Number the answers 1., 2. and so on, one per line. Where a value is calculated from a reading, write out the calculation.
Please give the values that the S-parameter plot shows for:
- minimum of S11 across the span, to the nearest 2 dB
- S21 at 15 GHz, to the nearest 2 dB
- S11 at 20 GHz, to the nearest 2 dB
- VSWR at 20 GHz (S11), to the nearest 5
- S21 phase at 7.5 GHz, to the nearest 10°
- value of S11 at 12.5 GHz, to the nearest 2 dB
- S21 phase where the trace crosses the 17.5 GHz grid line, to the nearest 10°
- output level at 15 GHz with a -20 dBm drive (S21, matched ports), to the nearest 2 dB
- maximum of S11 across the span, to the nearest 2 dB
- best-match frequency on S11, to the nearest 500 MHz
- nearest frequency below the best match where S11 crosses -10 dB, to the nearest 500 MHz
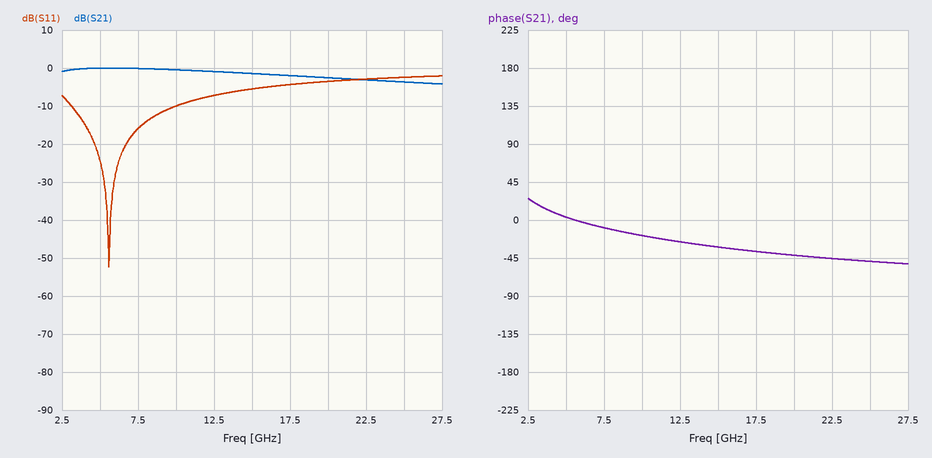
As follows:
1. -52 dB
2. -2 dB
3. -4 dB
4. |Γ| = 10^(-4/20) = 0.6310; VSWR = (1 + 0.6310)/(1 − 0.6310) ≈ 4.42, so 5 to the nearest 5
5. -10°
6. -8 dB
7. -40°
8. -20 dBm + (-2 dB) = -22 dBm
9. -2 dB
10. 5.5 GHz
11. 3.0 GHz
